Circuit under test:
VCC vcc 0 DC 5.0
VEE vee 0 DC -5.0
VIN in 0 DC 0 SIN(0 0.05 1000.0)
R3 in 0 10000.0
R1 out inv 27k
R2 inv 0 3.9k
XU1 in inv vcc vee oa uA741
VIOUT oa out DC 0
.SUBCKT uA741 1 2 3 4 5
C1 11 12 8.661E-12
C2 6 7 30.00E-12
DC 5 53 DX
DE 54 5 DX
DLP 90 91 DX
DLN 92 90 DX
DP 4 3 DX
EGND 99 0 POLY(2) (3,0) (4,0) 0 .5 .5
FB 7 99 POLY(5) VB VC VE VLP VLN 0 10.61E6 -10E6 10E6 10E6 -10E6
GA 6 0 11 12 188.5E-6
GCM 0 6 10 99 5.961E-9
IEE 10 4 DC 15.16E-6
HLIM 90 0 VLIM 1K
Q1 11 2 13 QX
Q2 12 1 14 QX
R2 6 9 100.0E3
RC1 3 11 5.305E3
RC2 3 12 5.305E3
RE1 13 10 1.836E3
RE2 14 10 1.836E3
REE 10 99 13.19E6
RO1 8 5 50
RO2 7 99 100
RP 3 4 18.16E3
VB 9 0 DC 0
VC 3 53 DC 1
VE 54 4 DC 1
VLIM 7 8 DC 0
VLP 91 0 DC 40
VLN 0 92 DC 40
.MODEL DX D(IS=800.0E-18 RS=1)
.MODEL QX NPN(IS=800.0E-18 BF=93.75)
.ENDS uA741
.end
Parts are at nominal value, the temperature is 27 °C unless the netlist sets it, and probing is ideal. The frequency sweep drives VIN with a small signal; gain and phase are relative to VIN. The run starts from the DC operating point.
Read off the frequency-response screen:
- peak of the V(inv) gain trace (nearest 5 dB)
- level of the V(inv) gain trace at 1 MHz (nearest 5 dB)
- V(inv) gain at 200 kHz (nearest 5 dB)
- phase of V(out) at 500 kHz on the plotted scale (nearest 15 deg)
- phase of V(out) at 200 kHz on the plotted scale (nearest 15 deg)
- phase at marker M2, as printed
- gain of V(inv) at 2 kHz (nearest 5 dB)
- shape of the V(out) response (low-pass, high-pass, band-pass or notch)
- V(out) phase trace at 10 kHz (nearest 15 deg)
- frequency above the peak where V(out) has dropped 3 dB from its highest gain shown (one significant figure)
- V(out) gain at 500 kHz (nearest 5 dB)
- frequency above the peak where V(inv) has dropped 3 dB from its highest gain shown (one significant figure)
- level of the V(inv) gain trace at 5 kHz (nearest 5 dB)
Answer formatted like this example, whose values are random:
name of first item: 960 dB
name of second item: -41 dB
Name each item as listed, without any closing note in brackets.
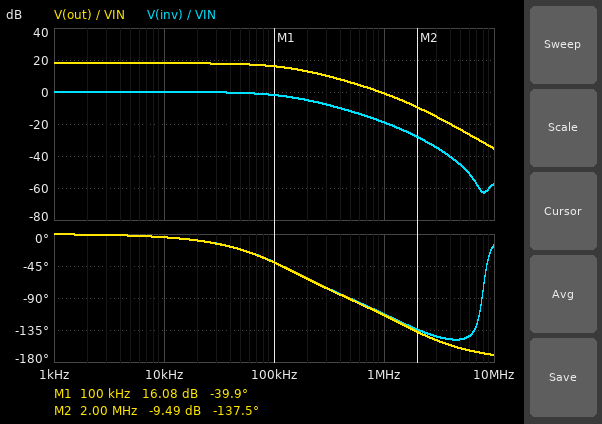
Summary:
peak of the V(inv) gain trace: 0 dB
level of the V(inv) gain trace at 1 MHz: -20 dB
V(inv) gain at 200 kHz: -5 dB
phase of V(out) at 500 kHz on the plotted scale: -90 deg
phase of V(out) at 200 kHz on the plotted scale: -60 deg
phase at marker M2, as printed: -137.5 deg
gain of V(inv) at 2 kHz: 0 dB
shape of the V(out) response: low-pass
V(out) phase trace at 10 kHz: 0 deg
frequency above the peak where V(out) has dropped 3 dB from its highest gain shown: 100 kHz
V(out) gain at 500 kHz: 5 dB
frequency above the peak where V(inv) has dropped 3 dB from its highest gain shown: 100 kHz
level of the V(inv) gain trace at 5 kHz: 0 dB
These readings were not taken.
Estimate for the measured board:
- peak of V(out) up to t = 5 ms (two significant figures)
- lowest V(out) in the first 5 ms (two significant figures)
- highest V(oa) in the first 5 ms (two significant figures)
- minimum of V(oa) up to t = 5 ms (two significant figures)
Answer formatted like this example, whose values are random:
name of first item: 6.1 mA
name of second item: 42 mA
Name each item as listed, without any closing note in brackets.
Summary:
peak of V(out) up to t = 5 ms: 400 mV
lowest V(out) in the first 5 ms: -390 mV
highest V(oa) in the first 5 ms: 400 mV
minimum of V(oa) up to t = 5 ms: -390 mV
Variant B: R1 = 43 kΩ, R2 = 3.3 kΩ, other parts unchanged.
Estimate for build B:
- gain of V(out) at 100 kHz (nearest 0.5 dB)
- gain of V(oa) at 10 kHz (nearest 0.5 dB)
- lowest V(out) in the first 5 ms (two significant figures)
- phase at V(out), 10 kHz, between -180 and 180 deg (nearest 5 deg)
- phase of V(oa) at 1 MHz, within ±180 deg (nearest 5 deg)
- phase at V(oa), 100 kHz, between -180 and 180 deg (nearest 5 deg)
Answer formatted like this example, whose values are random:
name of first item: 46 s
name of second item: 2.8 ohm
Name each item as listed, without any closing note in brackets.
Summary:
gain of V(out) at 100 kHz: 18.5 dB
gain of V(oa) at 10 kHz: 23.0 dB
lowest V(out) in the first 5 ms: -700 mV
phase at V(out), 10 kHz, between -180 and 180 deg: -10 deg
phase of V(oa) at 1 MHz, within ±180 deg: -115 deg
phase at V(oa), 100 kHz, between -180 and 180 deg: -55 deg
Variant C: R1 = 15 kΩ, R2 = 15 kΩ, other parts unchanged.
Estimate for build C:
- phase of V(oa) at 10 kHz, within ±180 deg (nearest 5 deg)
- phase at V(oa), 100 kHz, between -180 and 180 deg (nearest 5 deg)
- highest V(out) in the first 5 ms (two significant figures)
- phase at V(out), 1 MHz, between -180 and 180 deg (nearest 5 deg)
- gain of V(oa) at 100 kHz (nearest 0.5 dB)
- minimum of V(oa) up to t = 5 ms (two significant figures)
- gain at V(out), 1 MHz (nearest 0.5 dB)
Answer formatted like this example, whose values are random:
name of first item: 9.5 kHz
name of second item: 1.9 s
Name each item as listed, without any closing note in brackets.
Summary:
phase of V(oa) at 10 kHz, within ±180 deg: 0 deg
phase at V(oa), 100 kHz, between -180 and 180 deg: -10 deg
highest V(out) in the first 5 ms: 100 mV
phase at V(out), 1 MHz, between -180 and 180 deg: -95 deg
gain of V(oa) at 100 kHz: 6.0 dB
minimum of V(oa) up to t = 5 ms: -99 mV
gain at V(out), 1 MHz: 0 dB
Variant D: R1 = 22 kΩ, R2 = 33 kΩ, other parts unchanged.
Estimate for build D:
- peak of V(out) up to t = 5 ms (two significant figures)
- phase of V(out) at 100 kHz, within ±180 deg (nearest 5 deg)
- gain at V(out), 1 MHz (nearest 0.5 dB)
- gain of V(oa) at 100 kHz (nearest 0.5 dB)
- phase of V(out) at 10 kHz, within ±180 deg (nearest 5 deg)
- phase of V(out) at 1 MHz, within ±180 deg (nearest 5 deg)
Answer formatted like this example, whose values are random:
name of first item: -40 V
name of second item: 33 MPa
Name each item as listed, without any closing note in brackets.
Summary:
peak of V(out) up to t = 5 ms: 85 mV
phase of V(out) at 100 kHz, within ±180 deg: -10 deg
gain at V(out), 1 MHz: 0 dB
gain of V(oa) at 100 kHz: 4.5 dB
phase of V(out) at 10 kHz, within ±180 deg: 0 deg
phase of V(out) at 1 MHz, within ±180 deg: -90 deg
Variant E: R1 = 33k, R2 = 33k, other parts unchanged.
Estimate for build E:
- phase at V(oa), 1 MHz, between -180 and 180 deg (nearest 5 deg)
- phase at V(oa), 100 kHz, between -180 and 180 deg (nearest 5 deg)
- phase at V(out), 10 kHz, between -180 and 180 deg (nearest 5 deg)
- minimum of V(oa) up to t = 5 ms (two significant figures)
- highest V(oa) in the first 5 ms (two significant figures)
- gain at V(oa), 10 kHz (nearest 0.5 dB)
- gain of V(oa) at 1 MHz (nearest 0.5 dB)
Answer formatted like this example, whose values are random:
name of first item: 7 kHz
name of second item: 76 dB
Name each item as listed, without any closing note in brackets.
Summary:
phase at V(oa), 1 MHz, between -180 and 180 deg: -95 deg
phase at V(oa), 100 kHz, between -180 and 180 deg: -10 deg
phase at V(out), 10 kHz, between -180 and 180 deg: 0 deg
minimum of V(oa) up to t = 5 ms: -97 mV
highest V(oa) in the first 5 ms: 100 mV
gain at V(oa), 10 kHz: 6.0 dB
gain of V(oa) at 1 MHz: 0 dB
